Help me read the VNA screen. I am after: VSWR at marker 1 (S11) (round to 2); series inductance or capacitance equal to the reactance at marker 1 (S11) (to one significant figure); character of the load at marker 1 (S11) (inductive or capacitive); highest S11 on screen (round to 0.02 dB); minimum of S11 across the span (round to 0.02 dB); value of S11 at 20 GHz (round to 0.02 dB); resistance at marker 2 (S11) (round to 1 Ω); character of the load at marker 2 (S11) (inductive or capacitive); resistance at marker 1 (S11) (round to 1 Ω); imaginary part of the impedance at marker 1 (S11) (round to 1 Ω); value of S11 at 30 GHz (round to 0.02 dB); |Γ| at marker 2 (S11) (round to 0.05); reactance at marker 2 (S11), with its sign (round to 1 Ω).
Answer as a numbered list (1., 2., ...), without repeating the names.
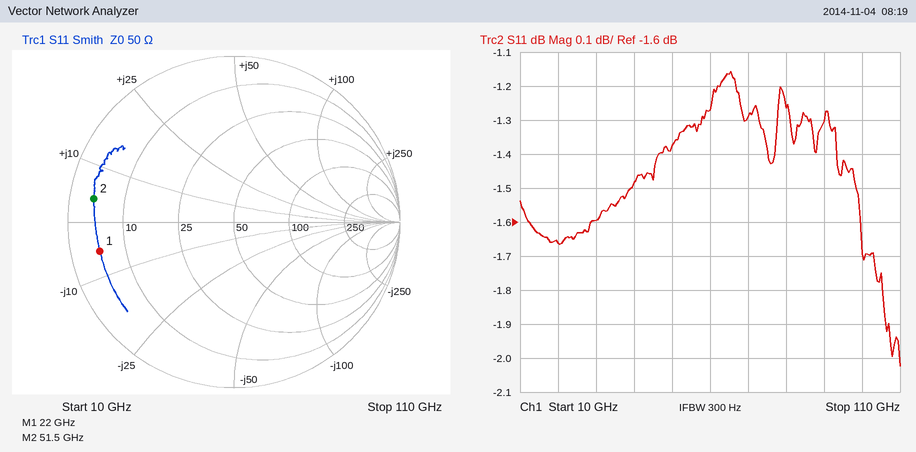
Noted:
1. 10
2. 1 pF
3. capacitive
4. -1.16 dB
5. -2.02 dB
6. -1.66 dB
7. 4 Ω
8. inductive
9. 5 Ω
10. -5 Ω
11. -1.60 dB
12. 0.85
13. +4 Ω
